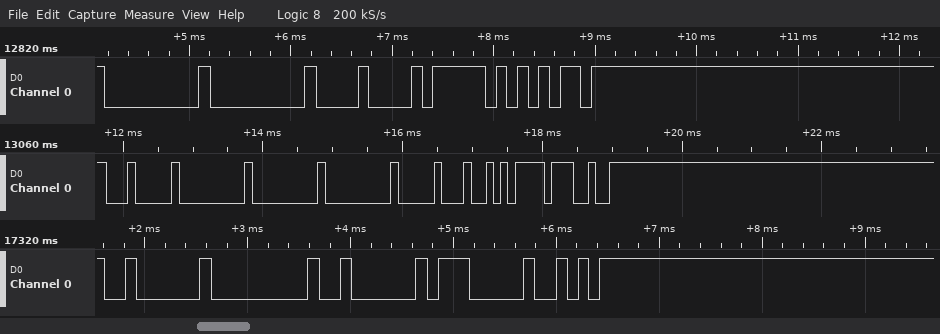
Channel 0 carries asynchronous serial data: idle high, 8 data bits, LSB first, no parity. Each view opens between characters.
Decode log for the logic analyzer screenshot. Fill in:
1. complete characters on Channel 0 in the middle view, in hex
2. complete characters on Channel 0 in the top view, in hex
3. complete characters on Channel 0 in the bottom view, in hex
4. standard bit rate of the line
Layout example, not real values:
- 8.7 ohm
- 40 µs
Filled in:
- 04, 00, 00, 00, 10, EA, 27
- 00, 00, 08, 5F, ED
- 02, 00, 02, 07, EA
- 9600 baud
